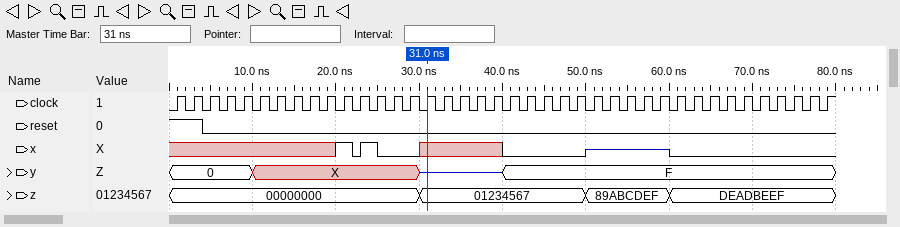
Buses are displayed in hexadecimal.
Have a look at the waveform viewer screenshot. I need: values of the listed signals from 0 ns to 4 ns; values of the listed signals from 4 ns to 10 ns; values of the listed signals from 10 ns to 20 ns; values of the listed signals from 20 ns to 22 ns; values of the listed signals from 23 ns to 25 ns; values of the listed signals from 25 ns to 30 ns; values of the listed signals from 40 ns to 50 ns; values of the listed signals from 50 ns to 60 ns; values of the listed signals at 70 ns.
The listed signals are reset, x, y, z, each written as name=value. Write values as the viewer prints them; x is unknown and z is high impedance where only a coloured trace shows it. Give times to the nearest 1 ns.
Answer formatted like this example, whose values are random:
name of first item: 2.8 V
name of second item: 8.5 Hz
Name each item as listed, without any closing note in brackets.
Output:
values of the listed signals from 0 ns to 4 ns: reset=1, x=x, y=0, z=00000000
values of the listed signals from 4 ns to 10 ns: reset=0, x=x, y=0, z=00000000
values of the listed signals from 10 ns to 20 ns: reset=0, x=x, y=X, z=00000000
values of the listed signals from 20 ns to 22 ns: reset=0, x=1, y=X, z=00000000
values of the listed signals from 23 ns to 25 ns: reset=0, x=1, y=X, z=00000000
values of the listed signals from 25 ns to 30 ns: reset=0, x=0, y=X, z=00000000
values of the listed signals from 40 ns to 50 ns: reset=0, x=0, y=F, z=01234567
values of the listed signals from 50 ns to 60 ns: reset=0, x=z, y=F, z=89ABCDEF
values of the listed signals at 70 ns: reset=0, x=0, y=F, z=DEADBEEF
